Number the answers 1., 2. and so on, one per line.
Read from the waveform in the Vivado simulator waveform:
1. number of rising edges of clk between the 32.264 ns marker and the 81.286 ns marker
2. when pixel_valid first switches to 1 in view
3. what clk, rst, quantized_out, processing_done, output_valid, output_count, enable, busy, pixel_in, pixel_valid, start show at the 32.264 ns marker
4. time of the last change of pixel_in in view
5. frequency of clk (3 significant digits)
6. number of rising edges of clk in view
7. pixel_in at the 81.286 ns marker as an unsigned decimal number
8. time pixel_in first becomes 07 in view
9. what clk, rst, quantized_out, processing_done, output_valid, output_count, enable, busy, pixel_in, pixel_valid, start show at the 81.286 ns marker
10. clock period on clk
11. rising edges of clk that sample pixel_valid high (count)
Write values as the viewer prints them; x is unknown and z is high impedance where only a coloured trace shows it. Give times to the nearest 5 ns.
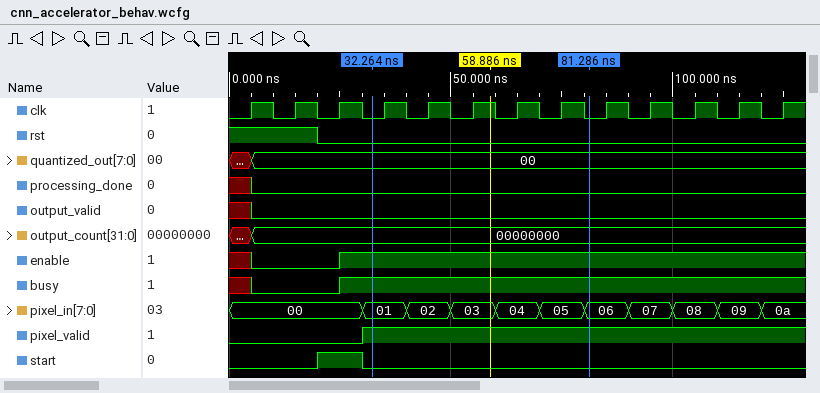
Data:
1. 5
2. 30 ns
3. clk=0, rst=0, quantized_out=00, processing_done=0, output_valid=0, output_count=00000000, enable=1, busy=1, pixel_in=01, pixel_valid=1, start=0
4. 120 ns
5. 100 MHz
6. 13
7. 6
8. 90 ns
9. clk=0, rst=0, quantized_out=00, processing_done=0, output_valid=0, output_count=00000000, enable=1, busy=1, pixel_in=06, pixel_valid=1, start=0
10. 10 ns
11. 10
